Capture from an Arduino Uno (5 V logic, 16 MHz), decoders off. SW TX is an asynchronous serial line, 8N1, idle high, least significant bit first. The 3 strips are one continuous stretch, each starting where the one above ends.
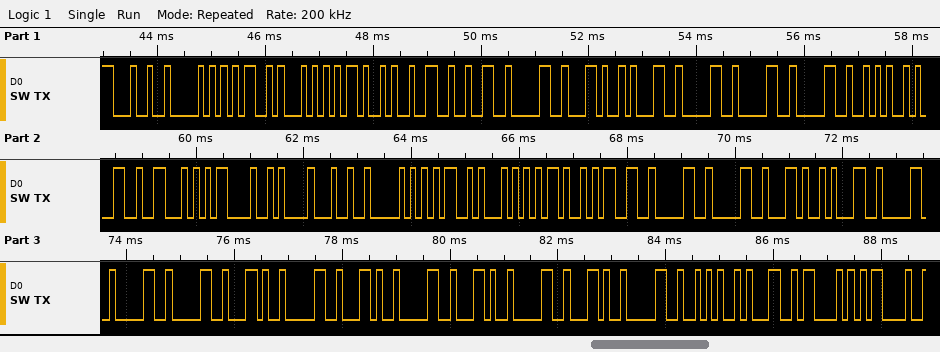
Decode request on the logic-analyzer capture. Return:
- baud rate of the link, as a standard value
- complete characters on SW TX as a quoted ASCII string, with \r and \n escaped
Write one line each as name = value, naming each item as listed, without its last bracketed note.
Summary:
baud rate of the link, as a standard value = 9600 baud
complete characters on SW TX as a quoted ASCII string, with \r and \n escaped = "$PMTK220,1000*1F\r\n$PMTK300,1000,0,0,0,0*1C\r"
